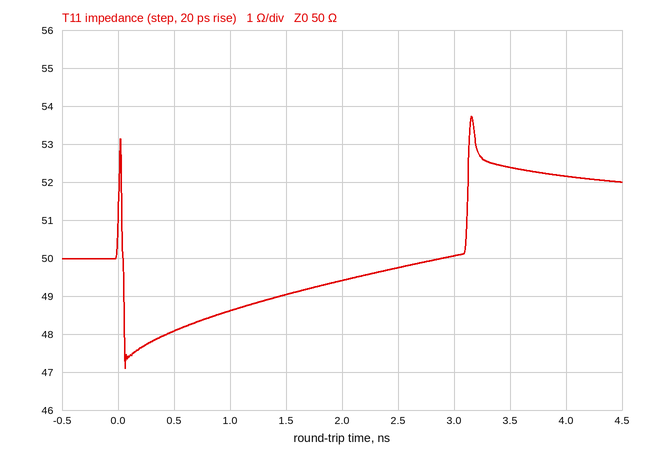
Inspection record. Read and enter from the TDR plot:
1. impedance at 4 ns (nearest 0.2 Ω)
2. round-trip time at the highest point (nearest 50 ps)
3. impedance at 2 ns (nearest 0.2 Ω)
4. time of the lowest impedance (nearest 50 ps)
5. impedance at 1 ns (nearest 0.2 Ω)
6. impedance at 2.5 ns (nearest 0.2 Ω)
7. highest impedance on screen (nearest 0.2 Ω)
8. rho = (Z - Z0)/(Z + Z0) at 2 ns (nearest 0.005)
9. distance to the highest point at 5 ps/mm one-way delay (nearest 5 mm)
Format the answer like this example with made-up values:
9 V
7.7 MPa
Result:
52.2 Ω
3.15 ns
49.4 Ω
50 ps
48.6 Ω
49.8 Ω
53.8 Ω
-0.005
315 mm
